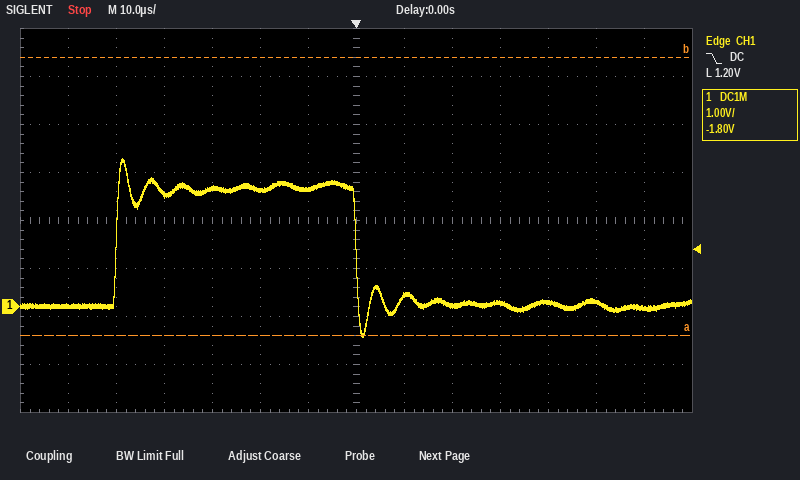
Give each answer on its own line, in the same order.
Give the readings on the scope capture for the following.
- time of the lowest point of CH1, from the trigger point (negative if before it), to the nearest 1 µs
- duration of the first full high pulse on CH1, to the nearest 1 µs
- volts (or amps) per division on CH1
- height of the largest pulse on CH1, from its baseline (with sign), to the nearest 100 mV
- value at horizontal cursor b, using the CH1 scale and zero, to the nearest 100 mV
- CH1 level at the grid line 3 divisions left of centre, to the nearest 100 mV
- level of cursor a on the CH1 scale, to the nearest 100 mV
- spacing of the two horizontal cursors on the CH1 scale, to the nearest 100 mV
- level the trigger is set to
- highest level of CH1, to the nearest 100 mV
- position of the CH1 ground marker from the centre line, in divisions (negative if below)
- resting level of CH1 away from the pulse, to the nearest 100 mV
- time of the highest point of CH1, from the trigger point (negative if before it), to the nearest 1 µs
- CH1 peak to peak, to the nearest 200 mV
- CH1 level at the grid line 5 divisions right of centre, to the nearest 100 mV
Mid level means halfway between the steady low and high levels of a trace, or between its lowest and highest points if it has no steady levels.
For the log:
+1 µs
50 µs
1 V
+3.1 V
5.2 V
2.5 V
-600 mV
5.8 V
1.20 V
3.1 V
-1.8 div
0.0 V
-49 µs
3.8 V
100 mV
